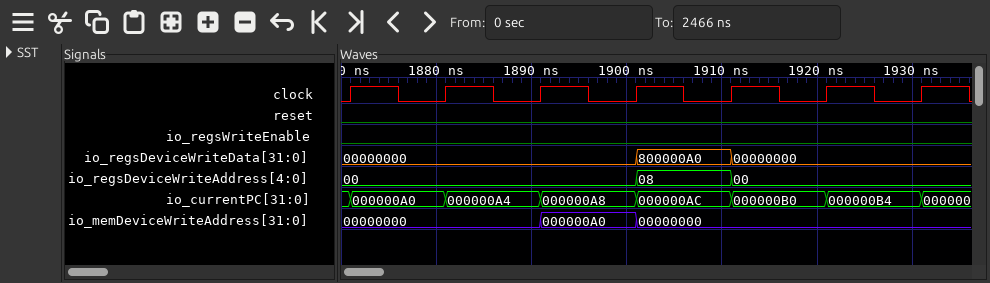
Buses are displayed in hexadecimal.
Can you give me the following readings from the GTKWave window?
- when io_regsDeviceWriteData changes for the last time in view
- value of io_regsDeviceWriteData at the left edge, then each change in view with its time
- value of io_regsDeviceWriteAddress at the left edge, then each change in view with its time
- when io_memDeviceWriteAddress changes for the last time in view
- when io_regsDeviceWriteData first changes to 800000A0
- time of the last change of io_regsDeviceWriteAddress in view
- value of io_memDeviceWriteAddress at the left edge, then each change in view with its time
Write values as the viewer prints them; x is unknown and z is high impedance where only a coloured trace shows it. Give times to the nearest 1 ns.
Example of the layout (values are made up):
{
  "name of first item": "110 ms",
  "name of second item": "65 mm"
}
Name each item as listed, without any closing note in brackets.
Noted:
{
  "when io_regsDeviceWriteData changes for the last time in view": "1911 ns",
  "value of io_regsDeviceWriteData at the left edge, then each change in view with its time": "00000000, 800000A0 at 1901 ns, 00000000 at 1911 ns",
  "value of io_regsDeviceWriteAddress at the left edge, then each change in view with its time": "00, 08 at 1901 ns, 00 at 1911 ns",
  "when io_memDeviceWriteAddress changes for the last time in view": "1901 ns",
  "when io_regsDeviceWriteData first changes to 800000A0": "1901 ns",
  "time of the last change of io_regsDeviceWriteAddress in view": "1911 ns",
  "value of io_memDeviceWriteAddress at the left edge, then each change in view with its time": "00000000, 000000A0 at 1891 ns, 00000000 at 1901 ns"
}
